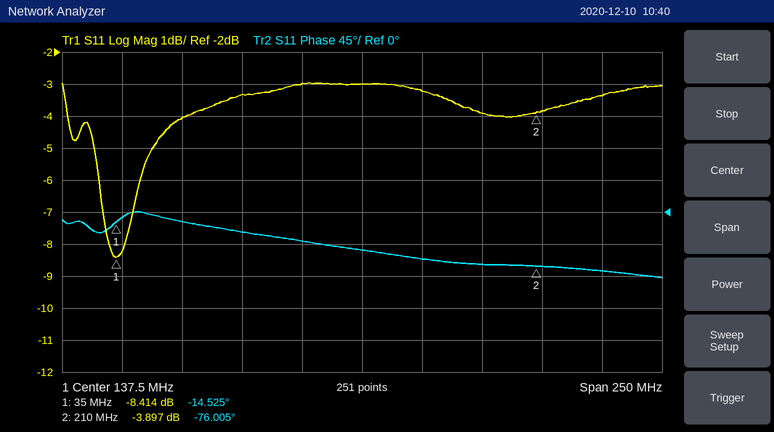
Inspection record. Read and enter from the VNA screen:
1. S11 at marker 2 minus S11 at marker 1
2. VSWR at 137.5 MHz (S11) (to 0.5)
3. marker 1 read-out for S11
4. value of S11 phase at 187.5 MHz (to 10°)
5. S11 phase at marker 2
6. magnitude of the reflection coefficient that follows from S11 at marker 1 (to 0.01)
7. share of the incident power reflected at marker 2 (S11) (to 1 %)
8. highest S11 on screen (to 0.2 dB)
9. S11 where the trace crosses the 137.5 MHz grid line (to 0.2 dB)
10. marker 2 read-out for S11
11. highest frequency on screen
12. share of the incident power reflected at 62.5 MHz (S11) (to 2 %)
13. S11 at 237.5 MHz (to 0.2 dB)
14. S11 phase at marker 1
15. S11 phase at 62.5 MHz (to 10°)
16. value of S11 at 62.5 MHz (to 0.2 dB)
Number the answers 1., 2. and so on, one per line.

1. 4.517 dB
2. 6.0
3. -8.414 dB
4. -70°
5. -76.005°
6. 0.38
7. 41 %
8. -3.0 dB
9. -3.0 dB
10. -3.897 dB
11. 262.5 MHz
12. 40 %
13. -3.4 dB
14. -14.525°
15. -10°
16. -4.0 dB
